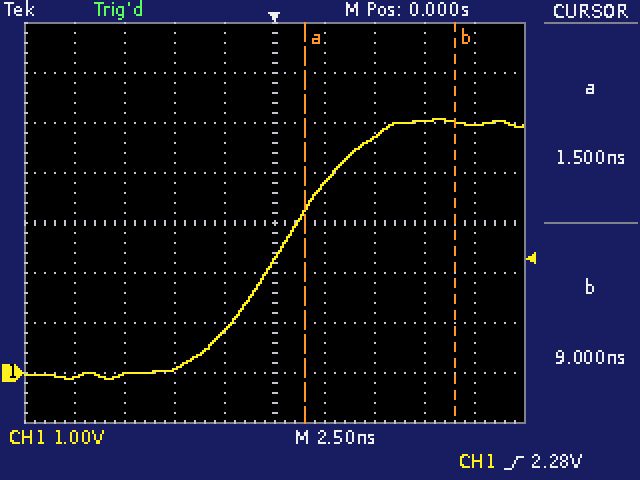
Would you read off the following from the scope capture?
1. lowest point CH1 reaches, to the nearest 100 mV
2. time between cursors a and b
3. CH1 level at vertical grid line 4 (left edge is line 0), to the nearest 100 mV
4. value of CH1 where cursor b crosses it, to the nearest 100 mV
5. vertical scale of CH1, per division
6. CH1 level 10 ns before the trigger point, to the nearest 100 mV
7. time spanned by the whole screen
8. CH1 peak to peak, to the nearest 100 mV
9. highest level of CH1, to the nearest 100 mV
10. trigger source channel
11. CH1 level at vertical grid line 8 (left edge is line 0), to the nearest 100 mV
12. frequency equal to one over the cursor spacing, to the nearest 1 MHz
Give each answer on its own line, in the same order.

-100 mV
7.50 ns
800 mV
5.0 V
1 V
-100 mV
25 ns
5.2 V
5.1 V
CH1
5.0 V
133 MHz
